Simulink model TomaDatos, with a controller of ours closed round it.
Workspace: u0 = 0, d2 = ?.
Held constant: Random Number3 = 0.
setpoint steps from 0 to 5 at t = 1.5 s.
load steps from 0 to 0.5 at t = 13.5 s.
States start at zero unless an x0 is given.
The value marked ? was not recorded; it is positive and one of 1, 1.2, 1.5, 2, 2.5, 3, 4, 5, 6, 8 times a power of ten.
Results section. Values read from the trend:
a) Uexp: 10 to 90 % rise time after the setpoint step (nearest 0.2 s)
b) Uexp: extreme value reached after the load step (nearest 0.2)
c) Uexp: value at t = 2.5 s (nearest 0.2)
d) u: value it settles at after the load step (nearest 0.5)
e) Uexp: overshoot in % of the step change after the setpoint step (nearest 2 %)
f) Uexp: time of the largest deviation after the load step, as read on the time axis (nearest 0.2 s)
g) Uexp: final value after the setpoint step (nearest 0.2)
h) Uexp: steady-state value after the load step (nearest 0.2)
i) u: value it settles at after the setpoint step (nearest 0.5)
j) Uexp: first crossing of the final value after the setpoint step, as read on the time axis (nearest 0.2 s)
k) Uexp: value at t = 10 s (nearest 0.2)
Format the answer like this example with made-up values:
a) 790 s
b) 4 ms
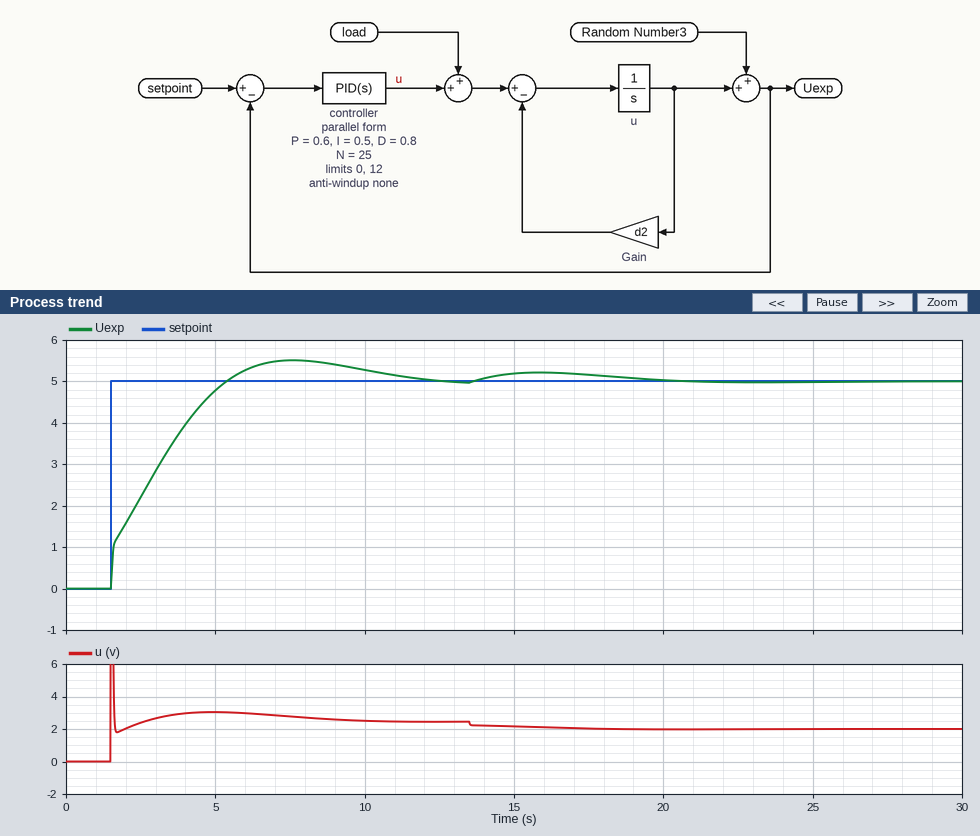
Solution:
a) 3.0 s
b) 5.2
c) 2.2
d) 2.0
e) 10 %
f) 15.8 s
g) 5.0
h) 5.0
i) 2.5
j) 5.4 s
k) 5.2
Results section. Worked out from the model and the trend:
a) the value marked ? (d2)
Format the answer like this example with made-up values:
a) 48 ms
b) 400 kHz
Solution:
a) 0.5
